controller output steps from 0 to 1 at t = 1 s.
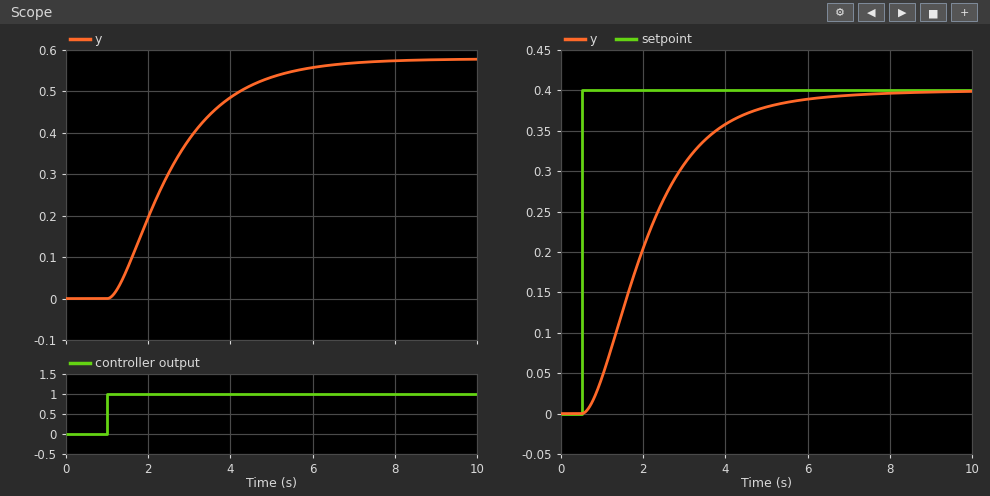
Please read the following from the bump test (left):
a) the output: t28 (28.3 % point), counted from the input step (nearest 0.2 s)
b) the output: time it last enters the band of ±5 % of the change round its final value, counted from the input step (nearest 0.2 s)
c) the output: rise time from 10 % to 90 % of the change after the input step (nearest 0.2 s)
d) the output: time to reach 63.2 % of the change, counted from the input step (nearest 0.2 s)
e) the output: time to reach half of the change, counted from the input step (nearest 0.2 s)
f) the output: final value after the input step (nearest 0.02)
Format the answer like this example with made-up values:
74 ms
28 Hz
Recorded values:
0.8 s
4.6 s
3.2 s
1.8 s
1.4 s
0.58
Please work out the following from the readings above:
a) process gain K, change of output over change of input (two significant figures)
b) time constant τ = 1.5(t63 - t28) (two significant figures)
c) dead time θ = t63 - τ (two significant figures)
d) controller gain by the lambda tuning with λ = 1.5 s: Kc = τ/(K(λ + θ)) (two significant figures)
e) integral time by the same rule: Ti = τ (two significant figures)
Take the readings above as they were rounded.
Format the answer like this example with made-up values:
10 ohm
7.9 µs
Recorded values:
0.58
1.5 s
0.30 s
1.4
1.5 s
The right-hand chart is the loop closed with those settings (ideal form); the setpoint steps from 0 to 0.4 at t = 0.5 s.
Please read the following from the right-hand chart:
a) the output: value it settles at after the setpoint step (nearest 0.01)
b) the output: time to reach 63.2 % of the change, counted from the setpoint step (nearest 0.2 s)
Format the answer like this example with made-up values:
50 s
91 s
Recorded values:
0.40
1.8 s
